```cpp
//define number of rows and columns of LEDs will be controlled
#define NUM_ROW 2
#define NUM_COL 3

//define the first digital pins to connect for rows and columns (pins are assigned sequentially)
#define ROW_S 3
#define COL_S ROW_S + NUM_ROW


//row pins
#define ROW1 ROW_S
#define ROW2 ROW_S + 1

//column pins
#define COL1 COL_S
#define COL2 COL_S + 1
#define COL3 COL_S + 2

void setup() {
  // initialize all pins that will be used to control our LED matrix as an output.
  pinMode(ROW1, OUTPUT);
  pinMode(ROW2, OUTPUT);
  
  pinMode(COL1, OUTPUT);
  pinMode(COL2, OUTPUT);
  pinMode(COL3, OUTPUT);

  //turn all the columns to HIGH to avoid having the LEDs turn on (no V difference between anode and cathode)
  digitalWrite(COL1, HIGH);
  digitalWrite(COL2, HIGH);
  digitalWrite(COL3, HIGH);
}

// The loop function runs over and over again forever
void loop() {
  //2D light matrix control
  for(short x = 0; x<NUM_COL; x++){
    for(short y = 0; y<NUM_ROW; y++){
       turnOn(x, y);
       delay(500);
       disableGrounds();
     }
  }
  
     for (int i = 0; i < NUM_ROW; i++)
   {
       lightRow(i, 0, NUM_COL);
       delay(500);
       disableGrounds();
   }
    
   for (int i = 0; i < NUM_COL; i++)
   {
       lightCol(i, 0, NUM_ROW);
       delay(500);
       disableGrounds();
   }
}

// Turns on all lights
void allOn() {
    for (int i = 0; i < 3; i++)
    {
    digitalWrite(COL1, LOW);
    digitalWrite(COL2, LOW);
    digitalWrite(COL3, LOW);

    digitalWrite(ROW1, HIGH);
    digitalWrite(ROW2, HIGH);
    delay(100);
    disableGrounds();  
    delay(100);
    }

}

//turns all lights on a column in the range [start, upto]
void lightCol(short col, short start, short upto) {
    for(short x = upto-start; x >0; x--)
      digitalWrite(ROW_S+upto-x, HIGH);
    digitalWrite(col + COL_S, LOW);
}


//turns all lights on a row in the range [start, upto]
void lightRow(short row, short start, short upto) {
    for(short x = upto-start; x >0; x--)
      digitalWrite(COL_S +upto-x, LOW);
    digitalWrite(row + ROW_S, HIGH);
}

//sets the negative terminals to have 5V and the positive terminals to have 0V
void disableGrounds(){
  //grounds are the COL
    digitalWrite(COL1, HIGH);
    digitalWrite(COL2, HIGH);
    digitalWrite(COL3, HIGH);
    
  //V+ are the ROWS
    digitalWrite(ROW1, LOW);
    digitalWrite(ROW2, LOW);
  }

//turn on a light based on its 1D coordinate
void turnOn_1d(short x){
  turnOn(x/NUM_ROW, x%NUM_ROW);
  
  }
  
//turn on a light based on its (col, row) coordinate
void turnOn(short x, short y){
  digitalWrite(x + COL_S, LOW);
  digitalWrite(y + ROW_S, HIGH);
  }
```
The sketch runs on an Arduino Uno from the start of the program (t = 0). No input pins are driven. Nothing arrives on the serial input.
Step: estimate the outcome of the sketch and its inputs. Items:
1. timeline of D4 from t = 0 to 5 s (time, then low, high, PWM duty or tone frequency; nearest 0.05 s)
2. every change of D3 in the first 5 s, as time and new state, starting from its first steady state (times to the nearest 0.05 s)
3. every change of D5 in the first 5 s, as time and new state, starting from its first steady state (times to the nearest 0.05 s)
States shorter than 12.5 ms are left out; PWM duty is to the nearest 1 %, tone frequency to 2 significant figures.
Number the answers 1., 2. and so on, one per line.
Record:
1. 0 s low; 0.5 s high; 1 s low; 1.5 s high; 2 s low; 2.5 s high; 3 s low; 3.5 s high
2. 0 s high; 0.5 s low; 1 s high; 1.5 s low; 2 s high; 2.5 s low; 3 s high; 3.5 s low; 4 s high
3. 0 s low; 1 s high; 3 s low; 4.5 s high
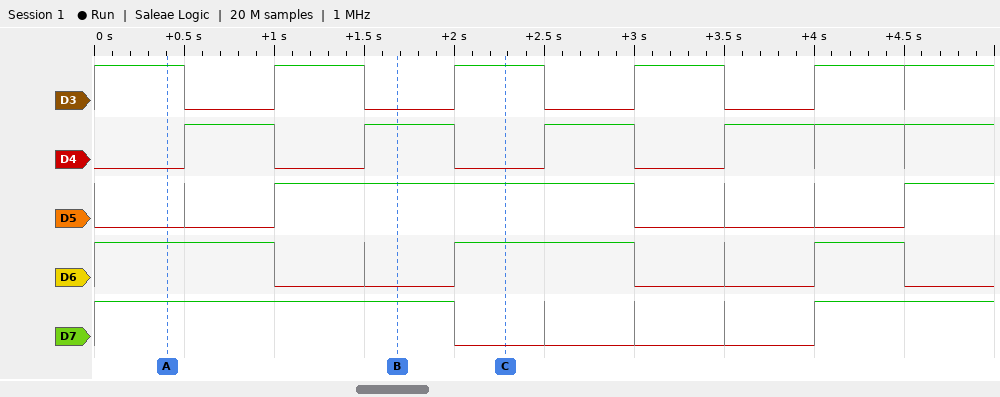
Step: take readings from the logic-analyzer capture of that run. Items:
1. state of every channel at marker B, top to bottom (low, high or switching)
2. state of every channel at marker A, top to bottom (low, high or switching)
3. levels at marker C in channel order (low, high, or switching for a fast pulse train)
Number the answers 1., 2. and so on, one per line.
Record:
1. D3 low, D4 high, D5 high, D6 low, D7 high
2. D3 high, D4 low, D5 low, D6 high, D7 high
3. D3 high, D4 low, D5 high, D6 high, D7 low
